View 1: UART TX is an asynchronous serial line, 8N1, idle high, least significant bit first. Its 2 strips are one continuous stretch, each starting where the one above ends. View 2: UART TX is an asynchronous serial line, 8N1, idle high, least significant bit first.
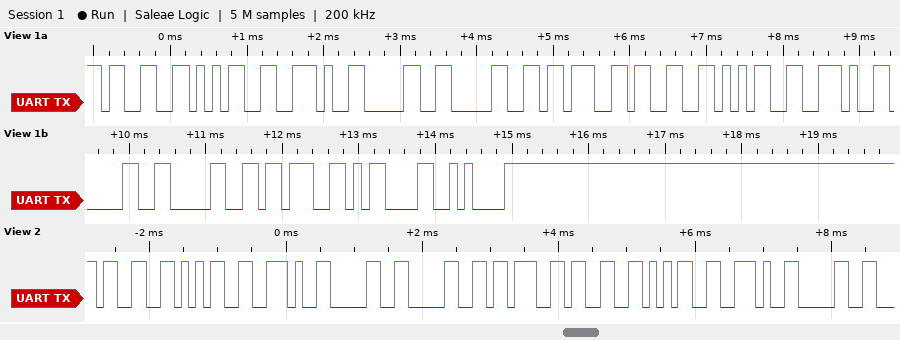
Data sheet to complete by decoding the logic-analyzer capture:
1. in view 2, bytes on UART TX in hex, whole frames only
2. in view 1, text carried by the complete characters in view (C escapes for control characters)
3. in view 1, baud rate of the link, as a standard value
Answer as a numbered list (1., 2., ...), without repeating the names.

1. 33 35 2E 30 30 3B 33 35 2E 30
2. "35.00;35.00;\r\n"
3. 9600 baud
